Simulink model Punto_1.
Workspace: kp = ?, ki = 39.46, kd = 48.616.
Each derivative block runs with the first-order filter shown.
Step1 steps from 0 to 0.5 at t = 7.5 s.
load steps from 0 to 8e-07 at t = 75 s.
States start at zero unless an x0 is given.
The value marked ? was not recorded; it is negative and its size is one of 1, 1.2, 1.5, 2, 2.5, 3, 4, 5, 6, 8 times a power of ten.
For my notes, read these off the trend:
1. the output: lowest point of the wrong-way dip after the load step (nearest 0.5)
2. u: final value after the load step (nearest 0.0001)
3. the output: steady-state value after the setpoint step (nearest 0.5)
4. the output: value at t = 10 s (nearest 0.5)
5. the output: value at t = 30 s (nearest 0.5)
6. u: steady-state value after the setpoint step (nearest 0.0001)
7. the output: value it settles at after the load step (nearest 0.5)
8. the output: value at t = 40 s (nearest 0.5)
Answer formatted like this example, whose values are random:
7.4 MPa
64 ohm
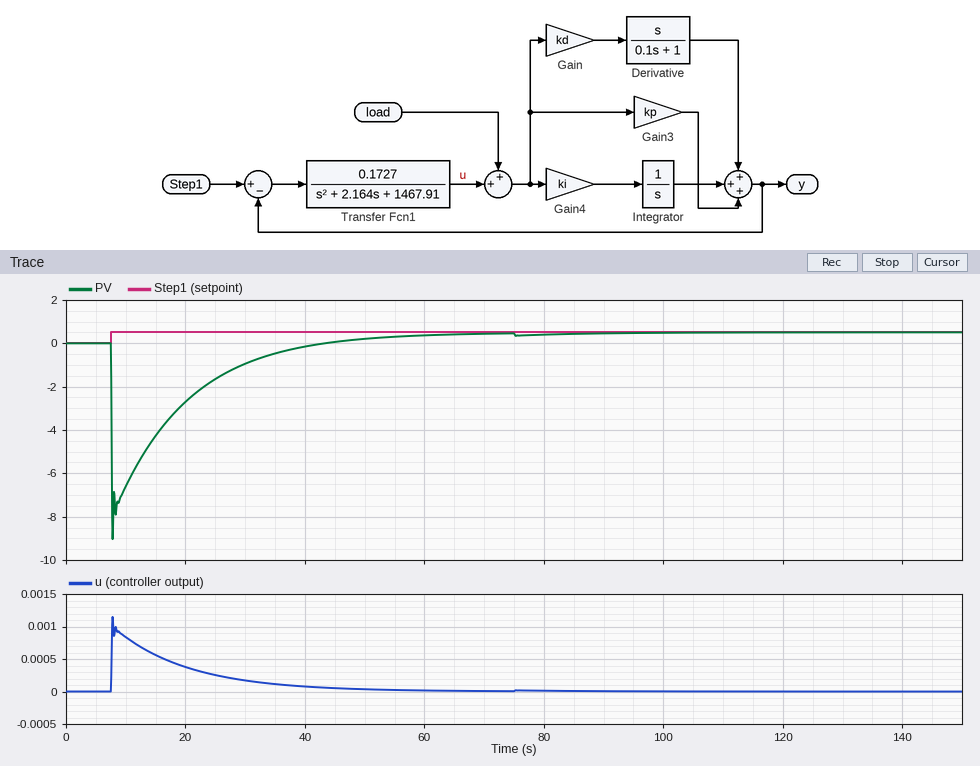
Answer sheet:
0.5
0.0000
0.5
-6.5
-1.0
0.0000
0.5
0.0
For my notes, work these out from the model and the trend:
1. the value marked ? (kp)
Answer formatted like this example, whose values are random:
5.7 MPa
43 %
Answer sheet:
-8000
